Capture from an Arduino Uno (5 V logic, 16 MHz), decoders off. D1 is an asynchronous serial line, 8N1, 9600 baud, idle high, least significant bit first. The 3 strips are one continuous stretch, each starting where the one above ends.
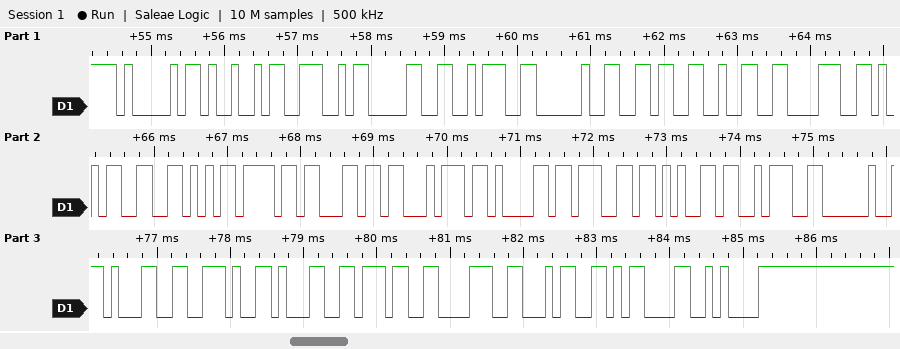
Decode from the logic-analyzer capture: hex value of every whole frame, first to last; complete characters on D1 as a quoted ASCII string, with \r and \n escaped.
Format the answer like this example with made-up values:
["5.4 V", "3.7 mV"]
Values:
["41 49 4E 30 3A 20 36 32 38 35 56 6F 6C 74 61 67 65 3A 20 31 2E 31 37 38 34 0D 0A", "\"AIN0: 6285Voltage: 1.1784\\r\\n\""]
